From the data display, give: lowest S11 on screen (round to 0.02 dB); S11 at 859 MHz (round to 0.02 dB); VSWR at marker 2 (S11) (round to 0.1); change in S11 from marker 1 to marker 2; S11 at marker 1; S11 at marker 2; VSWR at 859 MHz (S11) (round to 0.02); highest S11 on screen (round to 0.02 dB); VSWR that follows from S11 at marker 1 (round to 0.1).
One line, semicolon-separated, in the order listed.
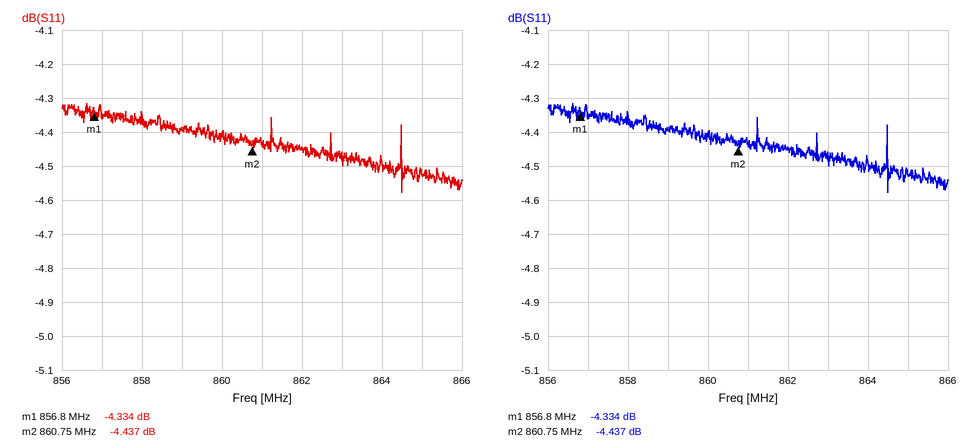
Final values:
-4.58 dB; -4.40 dB; 4.0; -0.103 dB; -4.334 dB; -4.437 dB; 4.04; -4.32 dB; 4.1
